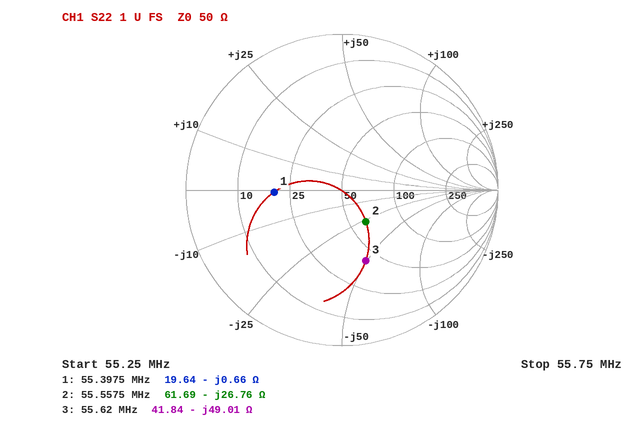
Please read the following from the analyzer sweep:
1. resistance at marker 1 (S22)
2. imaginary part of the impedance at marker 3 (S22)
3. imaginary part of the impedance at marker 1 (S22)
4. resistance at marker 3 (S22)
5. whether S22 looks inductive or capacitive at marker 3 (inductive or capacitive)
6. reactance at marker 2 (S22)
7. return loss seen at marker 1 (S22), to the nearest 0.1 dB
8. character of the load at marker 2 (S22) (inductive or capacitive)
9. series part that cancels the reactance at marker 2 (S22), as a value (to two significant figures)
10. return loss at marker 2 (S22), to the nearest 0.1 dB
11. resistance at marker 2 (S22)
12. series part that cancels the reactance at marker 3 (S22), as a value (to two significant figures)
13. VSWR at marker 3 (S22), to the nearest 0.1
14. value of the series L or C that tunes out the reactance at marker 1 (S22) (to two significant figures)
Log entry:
19.64 Ω
-49.01 Ω
-0.66 Ω
41.84 Ω
capacitive
-26.76 Ω
7.2 dB
capacitive
77 nH
11.9 dB
61.69 Ω
140 nH
2.8
1.9 nH
